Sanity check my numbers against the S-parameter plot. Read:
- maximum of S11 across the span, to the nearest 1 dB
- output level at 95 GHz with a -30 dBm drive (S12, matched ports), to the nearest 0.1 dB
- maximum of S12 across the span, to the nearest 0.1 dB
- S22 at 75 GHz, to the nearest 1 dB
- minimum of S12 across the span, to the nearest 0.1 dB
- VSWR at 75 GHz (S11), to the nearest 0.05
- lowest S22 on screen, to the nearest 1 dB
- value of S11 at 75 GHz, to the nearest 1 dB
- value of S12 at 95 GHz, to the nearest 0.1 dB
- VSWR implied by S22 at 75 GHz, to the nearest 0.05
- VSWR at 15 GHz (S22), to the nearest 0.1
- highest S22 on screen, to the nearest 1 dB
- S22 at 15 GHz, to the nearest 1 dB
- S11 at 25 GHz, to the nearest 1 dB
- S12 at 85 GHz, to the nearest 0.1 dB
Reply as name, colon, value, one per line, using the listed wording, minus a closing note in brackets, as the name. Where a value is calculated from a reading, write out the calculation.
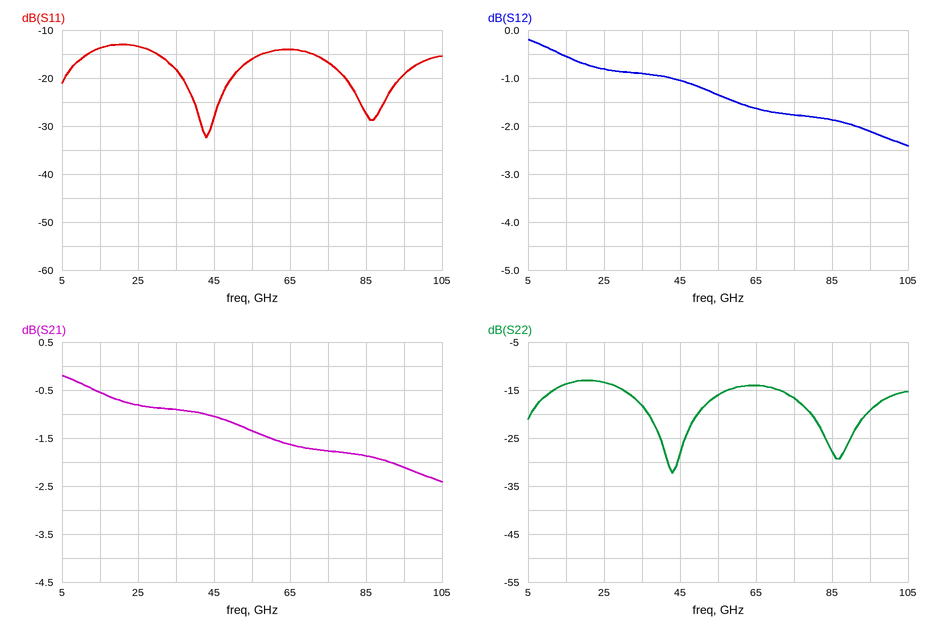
maximum of S11 across the span, to the nearest 1 dB: -13 dB
output level at 95 GHz with a -30 dBm drive (S12, matched ports), to the nearest 0.1 dB: -30 dBm + (-2.1 dB) = -32.1 dBm
maximum of S12 across the span, to the nearest 0.1 dB: -0.2 dB
S22 at 75 GHz, to the nearest 1 dB: -17 dB
minimum of S12 across the span, to the nearest 0.1 dB: -2.4 dB
VSWR at 75 GHz (S11), to the nearest 0.05: |Γ| = 10^(-17/20) = 0.1413; VSWR = (1 + 0.1413)/(1 − 0.1413) ≈ 1.33, so 1.35 to the nearest 0.05
lowest S22 on screen, to the nearest 1 dB: -32 dB
value of S11 at 75 GHz, to the nearest 1 dB: -17 dB
value of S12 at 95 GHz, to the nearest 0.1 dB: -2.1 dB
VSWR implied by S22 at 75 GHz, to the nearest 0.05: |Γ| = 10^(-17/20) = 0.1413; VSWR = (1 + 0.1413)/(1 − 0.1413) ≈ 1.33, so 1.35 to the nearest 0.05
VSWR at 15 GHz (S22), to the nearest 0.1: |Γ| = 10^(-14/20) = 0.1995; VSWR = (1 + 0.1995)/(1 − 0.1995) ≈ 1.5
highest S22 on screen, to the nearest 1 dB: -13 dB
S22 at 15 GHz, to the nearest 1 dB: -14 dB
S11 at 25 GHz, to the nearest 1 dB: -13 dB
S12 at 85 GHz, to the nearest 0.1 dB: -1.9 dB
